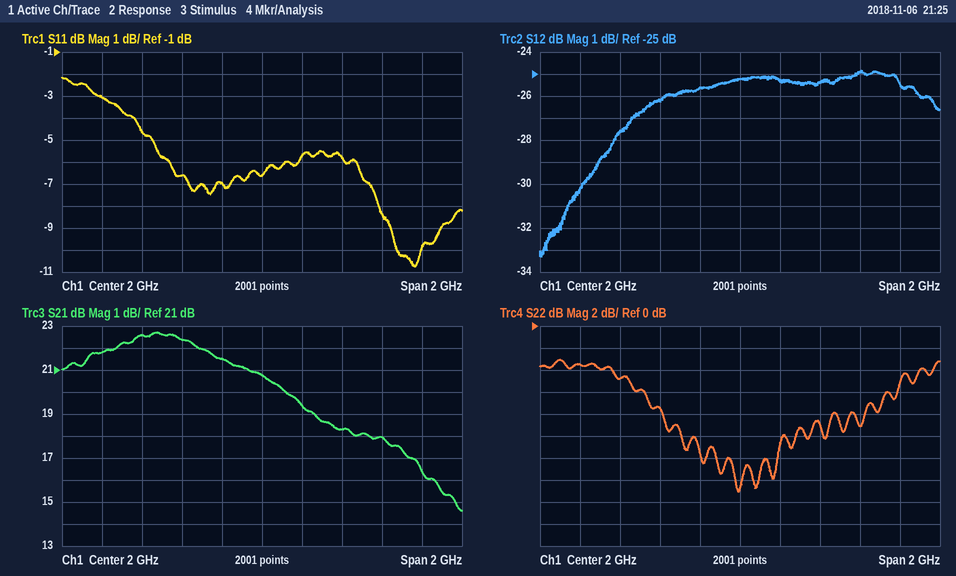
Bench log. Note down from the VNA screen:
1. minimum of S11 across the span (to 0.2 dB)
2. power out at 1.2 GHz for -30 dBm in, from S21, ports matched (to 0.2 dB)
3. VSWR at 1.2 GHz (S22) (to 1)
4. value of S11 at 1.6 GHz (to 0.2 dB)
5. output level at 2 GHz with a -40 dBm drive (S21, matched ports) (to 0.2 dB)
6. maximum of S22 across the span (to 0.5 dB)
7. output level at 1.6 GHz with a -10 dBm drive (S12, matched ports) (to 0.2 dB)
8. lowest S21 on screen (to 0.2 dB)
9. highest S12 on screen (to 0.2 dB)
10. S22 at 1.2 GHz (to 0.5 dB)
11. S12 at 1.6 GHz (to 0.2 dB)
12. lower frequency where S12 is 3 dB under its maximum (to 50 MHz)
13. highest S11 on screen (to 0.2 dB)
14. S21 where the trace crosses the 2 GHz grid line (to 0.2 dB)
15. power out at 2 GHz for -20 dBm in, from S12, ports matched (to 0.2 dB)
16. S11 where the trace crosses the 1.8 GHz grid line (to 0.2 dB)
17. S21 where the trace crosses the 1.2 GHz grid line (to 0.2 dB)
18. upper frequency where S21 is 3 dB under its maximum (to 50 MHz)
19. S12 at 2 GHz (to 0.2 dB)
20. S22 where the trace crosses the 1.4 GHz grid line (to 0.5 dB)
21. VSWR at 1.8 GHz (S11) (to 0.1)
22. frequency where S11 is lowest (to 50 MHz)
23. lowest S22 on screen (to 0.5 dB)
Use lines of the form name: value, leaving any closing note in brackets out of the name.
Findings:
minimum of S11 across the span: -10.8 dB
power out at 1.2 GHz for -30 dBm in, from S21, ports matched: -8.2 dBm
VSWR at 1.2 GHz (S22): 5
value of S11 at 1.6 GHz: -6.6 dB
output level at 2 GHz with a -40 dBm drive (S21, matched ports): -19.2 dBm
maximum of S22 across the span: -3.0 dB
output level at 1.6 GHz with a -10 dBm drive (S12, matched ports): -36.2 dBm
lowest S21 on screen: 14.6 dB
highest S12 on screen: -24.8 dB
S22 at 1.2 GHz: -3.5 dB
S12 at 1.6 GHz: -26.2 dB
lower frequency where S12 is 3 dB under its maximum: 1.40 GHz
highest S11 on screen: -2.2 dB
S21 where the trace crosses the 2 GHz grid line: 20.8 dB
power out at 2 GHz for -20 dBm in, from S12, ports matched: -45.2 dBm
S11 where the trace crosses the 1.8 GHz grid line: -7.0 dB
S21 where the trace crosses the 1.2 GHz grid line: 21.8 dB
upper frequency where S21 is 3 dB under its maximum: 2.15 GHz
S12 at 2 GHz: -25.2 dB
S22 where the trace crosses the 1.4 GHz grid line: -5.0 dB
VSWR at 1.8 GHz (S11): 2.6
frequency where S11 is lowest: 2.75 GHz
lowest S22 on screen: -15.0 dB
